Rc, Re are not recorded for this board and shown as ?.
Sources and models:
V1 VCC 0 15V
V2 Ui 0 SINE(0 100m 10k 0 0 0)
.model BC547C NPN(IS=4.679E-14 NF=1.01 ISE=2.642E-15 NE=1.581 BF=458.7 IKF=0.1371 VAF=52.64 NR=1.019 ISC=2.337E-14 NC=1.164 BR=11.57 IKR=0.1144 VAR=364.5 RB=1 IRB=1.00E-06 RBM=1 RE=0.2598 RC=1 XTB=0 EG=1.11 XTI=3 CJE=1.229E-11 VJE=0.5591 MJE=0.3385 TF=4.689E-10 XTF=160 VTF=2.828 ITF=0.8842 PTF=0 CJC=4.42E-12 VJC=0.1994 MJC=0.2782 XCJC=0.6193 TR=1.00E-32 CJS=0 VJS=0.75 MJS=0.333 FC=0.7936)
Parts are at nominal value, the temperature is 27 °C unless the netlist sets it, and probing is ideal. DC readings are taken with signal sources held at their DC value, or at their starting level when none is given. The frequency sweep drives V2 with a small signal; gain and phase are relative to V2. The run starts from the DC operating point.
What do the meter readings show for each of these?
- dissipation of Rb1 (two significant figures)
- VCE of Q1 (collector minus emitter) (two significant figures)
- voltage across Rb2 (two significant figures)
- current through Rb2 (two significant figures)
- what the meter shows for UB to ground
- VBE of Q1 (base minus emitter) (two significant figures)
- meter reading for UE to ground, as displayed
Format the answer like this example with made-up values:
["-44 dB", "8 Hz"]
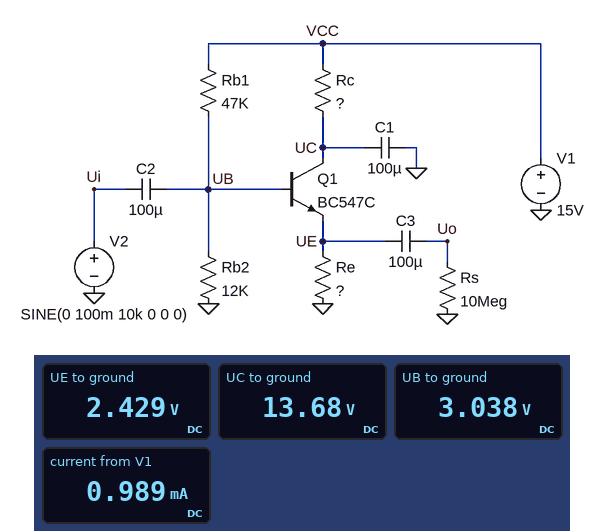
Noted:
["3.0 mW", "11 V", "3.0 V", "250 µA", "3.038 V", "610 mV", "2.429 V"]
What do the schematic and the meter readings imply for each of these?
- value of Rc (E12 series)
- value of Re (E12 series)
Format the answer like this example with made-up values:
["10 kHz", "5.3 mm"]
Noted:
["1.8 kΩ", "3.3 kΩ"]
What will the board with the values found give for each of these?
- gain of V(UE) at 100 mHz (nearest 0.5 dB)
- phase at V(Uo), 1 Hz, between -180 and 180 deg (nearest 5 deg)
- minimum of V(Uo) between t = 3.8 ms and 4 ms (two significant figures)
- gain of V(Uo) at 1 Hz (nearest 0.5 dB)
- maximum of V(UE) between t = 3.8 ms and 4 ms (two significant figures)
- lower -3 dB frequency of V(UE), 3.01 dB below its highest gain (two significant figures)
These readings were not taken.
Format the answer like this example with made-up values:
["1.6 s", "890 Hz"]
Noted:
["-6.0 dB", "10 deg", "-99 mV", "0 dB", "2.5 V", "170 mHz"]
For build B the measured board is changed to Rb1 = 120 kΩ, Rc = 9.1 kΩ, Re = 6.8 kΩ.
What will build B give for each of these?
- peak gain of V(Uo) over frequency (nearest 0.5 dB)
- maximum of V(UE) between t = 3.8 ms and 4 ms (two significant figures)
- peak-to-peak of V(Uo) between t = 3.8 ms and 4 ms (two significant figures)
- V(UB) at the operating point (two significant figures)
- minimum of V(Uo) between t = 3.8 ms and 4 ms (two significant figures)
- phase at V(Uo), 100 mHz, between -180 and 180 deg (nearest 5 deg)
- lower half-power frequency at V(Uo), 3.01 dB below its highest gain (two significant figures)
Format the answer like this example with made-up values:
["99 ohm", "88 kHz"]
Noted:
["-0.5 dB", "900 mV", "190 mV", "1.4 V", "-97 mV", "55 deg", "150 mHz"]
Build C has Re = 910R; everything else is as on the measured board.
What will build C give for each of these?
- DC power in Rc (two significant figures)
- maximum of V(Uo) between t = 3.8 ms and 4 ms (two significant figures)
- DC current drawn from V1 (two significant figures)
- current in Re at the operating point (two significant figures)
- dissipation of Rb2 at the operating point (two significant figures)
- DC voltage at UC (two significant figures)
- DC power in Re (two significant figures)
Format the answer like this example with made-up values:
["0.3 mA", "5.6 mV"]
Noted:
["12 mW", "99 mV", "2.8 mA", "2.6 mA", "750 µW", "10 V", "6.1 mW"]
